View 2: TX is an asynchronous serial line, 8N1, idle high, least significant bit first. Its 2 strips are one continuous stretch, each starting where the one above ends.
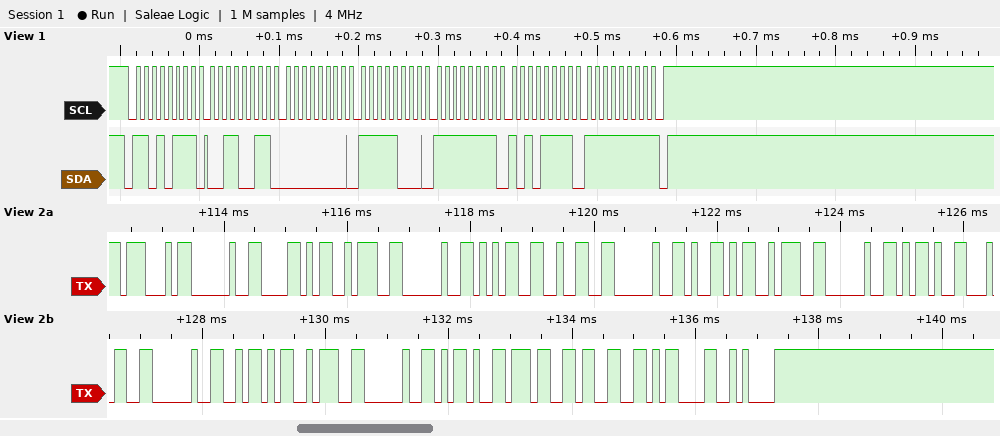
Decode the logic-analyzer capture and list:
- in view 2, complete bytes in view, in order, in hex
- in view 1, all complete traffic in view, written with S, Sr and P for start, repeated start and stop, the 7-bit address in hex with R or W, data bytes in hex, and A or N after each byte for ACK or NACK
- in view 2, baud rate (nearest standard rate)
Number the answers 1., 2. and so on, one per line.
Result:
1. 47 20 58 3A 20 35 32 20 59 3A 20 2D 34 20 5A 3A 20 2D 37 33 0D 0A
2. S 6BR A 33 A 00 A F8 A FF A AF A FF N P
3. 9600 baud
